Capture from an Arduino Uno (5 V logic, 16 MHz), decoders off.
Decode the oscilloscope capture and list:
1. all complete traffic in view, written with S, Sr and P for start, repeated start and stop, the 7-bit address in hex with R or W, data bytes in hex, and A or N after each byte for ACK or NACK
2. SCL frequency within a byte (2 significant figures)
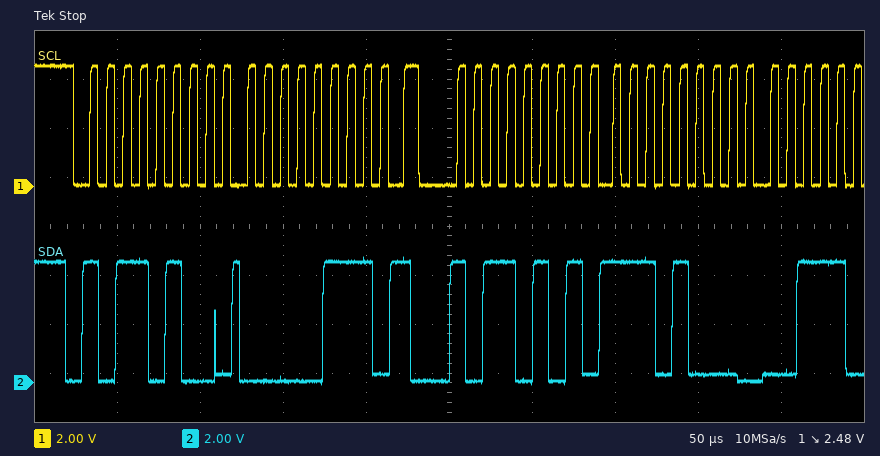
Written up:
S 5AW A 07 A Sr 5AR A E8 A
100 kHz
